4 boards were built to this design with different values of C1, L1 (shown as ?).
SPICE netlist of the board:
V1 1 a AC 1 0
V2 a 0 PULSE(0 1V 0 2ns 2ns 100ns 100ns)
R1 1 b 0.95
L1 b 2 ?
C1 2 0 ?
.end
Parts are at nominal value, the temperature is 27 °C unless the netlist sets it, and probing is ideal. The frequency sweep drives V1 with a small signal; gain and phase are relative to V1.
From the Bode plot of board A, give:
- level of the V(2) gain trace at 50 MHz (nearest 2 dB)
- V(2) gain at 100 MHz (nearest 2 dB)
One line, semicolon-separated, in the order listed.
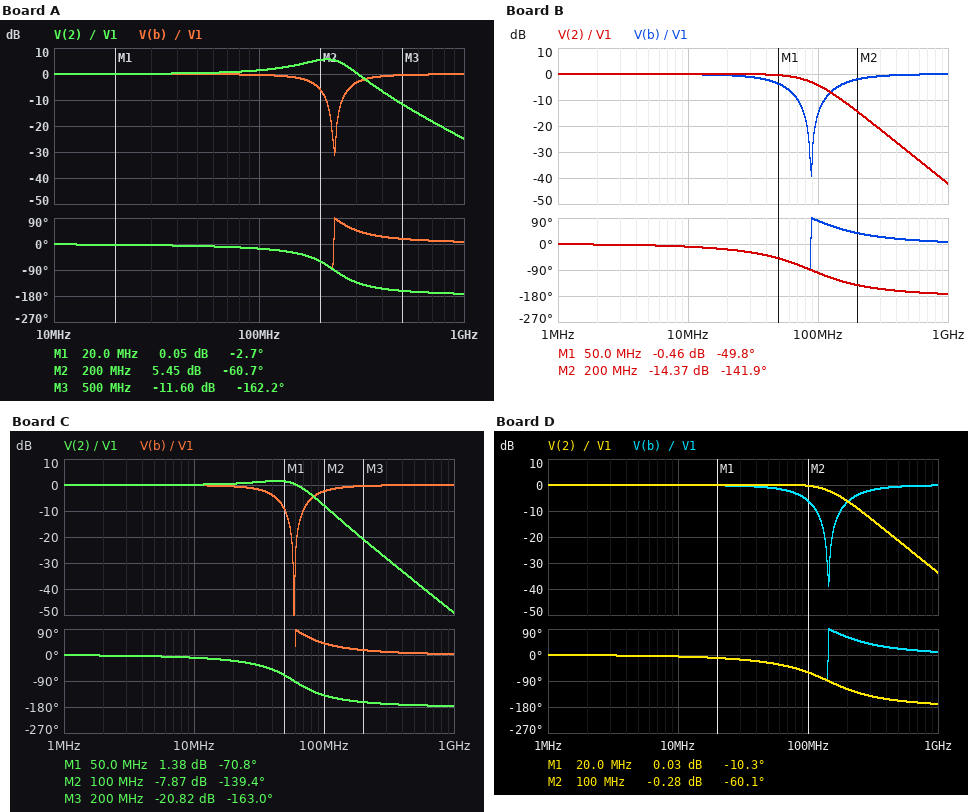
0 dB; 2 dB
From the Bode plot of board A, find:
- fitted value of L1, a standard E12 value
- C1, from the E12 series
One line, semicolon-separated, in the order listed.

1.2 nH; 390 pF
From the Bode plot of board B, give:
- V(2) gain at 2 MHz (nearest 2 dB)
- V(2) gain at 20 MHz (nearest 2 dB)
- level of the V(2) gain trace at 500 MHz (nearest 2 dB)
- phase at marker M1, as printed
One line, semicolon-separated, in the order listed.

0 dB; 0 dB; -30 dB; -49.8 deg
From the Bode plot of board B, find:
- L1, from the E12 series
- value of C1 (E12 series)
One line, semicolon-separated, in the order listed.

1.2 nH; 2.7 nF
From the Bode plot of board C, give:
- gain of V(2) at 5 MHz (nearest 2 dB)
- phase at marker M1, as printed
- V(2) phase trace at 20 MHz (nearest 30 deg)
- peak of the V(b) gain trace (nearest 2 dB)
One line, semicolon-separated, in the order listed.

0 dB; -70.8 deg; -30 deg; 0 dB
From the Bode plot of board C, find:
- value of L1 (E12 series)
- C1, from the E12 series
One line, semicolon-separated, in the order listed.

2.7 nH; 2.7 nF
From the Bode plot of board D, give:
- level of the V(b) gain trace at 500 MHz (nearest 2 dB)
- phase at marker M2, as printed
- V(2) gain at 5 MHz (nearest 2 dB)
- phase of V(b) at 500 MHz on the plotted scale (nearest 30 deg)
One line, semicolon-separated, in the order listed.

0 dB; -60.1 deg; 0 dB; 30 deg
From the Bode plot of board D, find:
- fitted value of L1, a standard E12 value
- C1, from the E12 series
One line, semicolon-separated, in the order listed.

820 pH; 1.5 nF
